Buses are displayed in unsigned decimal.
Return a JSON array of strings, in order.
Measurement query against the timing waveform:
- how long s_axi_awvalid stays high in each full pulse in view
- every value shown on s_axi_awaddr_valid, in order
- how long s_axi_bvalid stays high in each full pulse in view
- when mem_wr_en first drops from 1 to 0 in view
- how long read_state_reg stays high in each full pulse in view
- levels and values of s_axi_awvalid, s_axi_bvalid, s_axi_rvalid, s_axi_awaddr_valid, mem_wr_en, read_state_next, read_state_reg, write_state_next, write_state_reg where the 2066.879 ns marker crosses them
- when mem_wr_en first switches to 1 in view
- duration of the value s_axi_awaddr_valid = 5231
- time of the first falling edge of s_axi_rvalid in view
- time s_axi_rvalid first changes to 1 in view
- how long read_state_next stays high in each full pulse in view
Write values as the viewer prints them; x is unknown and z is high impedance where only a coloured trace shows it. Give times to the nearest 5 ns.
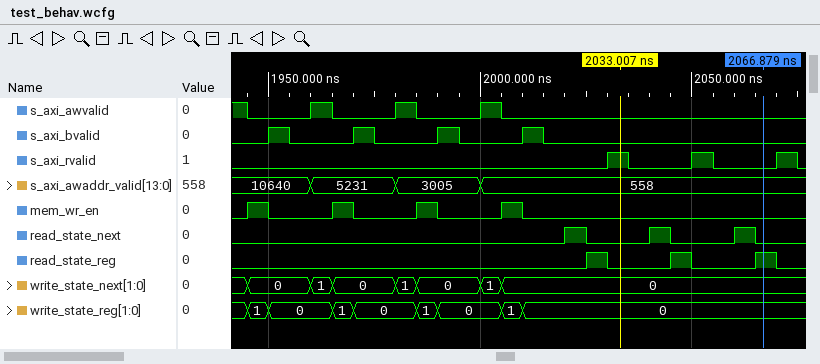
["5 ns, 5 ns, 5 ns", "10640, 5231, 3005, 558", "5 ns, 5 ns, 5 ns, 5 ns", "1950 ns", "5 ns, 5 ns, 5 ns", "s_axi_awvalid=0, s_axi_bvalid=0, s_axi_rvalid=0, s_axi_awaddr_valid=558, mem_wr_en=0, read_state_next=0, read_state_reg=1, write_state_next=0, write_state_reg=0", "1945 ns", "20 ns", "2035 ns", "2030 ns", "5 ns, 5 ns, 5 ns"]
